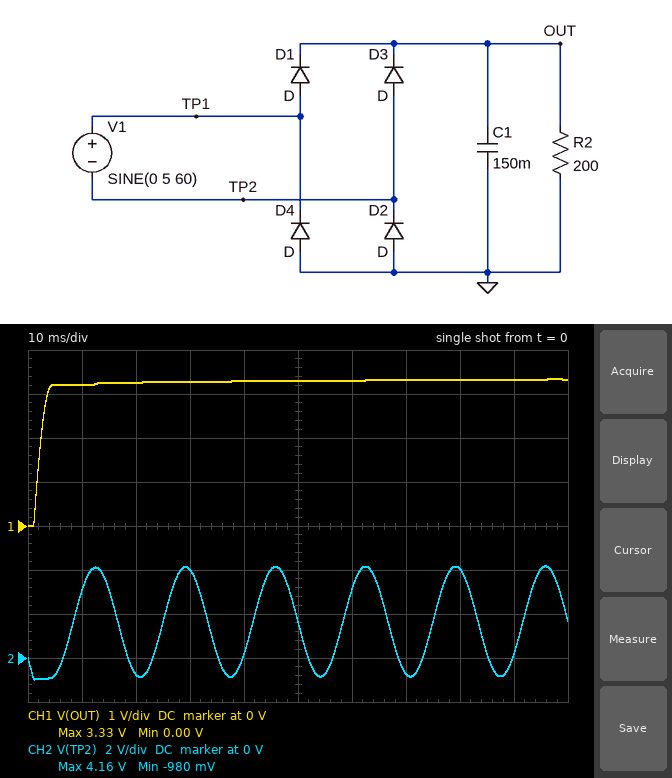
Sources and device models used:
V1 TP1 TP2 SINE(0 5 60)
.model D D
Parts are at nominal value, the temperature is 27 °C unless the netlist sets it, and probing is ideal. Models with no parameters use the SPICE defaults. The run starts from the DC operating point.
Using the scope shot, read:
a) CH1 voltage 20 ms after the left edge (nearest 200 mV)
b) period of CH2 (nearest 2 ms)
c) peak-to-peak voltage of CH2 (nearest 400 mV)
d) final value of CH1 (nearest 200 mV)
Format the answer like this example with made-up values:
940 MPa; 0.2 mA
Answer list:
3.2 V; 16 ms; 5.2 V; 3.4 V
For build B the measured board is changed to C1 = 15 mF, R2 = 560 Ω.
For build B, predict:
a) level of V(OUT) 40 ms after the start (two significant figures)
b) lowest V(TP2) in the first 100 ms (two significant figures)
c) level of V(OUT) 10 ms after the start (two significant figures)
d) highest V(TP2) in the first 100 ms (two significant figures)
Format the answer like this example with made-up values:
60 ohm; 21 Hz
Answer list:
3.4 V; -920 mV; 3.3 V; 4.2 V
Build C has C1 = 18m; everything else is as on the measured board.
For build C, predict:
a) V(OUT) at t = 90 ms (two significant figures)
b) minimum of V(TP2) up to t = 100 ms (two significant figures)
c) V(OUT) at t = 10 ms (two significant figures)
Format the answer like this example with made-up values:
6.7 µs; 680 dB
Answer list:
3.4 V; -920 mV; 3.3 V
